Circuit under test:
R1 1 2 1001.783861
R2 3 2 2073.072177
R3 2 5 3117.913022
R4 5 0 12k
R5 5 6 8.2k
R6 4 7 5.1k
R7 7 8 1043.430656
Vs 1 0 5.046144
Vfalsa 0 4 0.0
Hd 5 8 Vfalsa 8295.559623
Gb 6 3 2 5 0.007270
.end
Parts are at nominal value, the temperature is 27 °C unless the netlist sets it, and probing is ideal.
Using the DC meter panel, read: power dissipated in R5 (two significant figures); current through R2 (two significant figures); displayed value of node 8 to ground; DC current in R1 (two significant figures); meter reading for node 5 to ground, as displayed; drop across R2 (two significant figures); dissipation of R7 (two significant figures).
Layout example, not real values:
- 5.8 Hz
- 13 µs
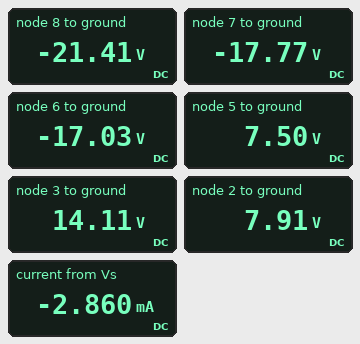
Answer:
- 73 mW
- 3.0 mA
- -21.41 V
- 2.9 mA
- 7.50 V
- 6.2 V
- 13 mW
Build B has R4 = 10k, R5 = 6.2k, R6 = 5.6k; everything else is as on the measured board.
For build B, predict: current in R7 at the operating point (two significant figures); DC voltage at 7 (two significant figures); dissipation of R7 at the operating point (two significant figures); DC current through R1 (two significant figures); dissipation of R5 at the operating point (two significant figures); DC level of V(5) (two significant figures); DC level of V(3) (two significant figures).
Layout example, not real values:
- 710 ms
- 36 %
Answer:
- 5.4 mA
- -30 V
- 30 mW
- 4.5 mA
- 140 mW
- 8.9 V
- 19 V
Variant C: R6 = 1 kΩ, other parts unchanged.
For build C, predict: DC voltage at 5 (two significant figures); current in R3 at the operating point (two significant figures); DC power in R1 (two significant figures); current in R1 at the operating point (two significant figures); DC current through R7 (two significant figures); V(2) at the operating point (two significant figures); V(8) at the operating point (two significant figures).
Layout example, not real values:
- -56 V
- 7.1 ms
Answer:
- 5.4 V
- 19 µA
- 170 µW
- 410 µA
- 860 µA
- 5.5 V
- -1.8 V
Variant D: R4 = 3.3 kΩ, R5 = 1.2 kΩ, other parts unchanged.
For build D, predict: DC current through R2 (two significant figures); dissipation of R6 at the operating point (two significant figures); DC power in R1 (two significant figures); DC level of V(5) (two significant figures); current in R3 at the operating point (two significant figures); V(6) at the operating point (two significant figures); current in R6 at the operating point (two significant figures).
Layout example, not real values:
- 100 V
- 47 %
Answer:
- 990 µA
- 38 mW
- 900 µW
- 5.9 V
- 44 µA
- 4.7 V
- 2.7 mA
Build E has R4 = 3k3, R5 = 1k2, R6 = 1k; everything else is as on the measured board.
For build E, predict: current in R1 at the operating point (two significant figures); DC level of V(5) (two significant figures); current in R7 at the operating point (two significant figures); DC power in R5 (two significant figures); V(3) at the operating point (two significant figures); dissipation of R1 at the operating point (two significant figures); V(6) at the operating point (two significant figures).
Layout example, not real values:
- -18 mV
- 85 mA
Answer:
- 640 µA
- 4.5 V
- 720 µA
- 540 µW
- 3.0 V
- 410 µW
- 5.3 V
